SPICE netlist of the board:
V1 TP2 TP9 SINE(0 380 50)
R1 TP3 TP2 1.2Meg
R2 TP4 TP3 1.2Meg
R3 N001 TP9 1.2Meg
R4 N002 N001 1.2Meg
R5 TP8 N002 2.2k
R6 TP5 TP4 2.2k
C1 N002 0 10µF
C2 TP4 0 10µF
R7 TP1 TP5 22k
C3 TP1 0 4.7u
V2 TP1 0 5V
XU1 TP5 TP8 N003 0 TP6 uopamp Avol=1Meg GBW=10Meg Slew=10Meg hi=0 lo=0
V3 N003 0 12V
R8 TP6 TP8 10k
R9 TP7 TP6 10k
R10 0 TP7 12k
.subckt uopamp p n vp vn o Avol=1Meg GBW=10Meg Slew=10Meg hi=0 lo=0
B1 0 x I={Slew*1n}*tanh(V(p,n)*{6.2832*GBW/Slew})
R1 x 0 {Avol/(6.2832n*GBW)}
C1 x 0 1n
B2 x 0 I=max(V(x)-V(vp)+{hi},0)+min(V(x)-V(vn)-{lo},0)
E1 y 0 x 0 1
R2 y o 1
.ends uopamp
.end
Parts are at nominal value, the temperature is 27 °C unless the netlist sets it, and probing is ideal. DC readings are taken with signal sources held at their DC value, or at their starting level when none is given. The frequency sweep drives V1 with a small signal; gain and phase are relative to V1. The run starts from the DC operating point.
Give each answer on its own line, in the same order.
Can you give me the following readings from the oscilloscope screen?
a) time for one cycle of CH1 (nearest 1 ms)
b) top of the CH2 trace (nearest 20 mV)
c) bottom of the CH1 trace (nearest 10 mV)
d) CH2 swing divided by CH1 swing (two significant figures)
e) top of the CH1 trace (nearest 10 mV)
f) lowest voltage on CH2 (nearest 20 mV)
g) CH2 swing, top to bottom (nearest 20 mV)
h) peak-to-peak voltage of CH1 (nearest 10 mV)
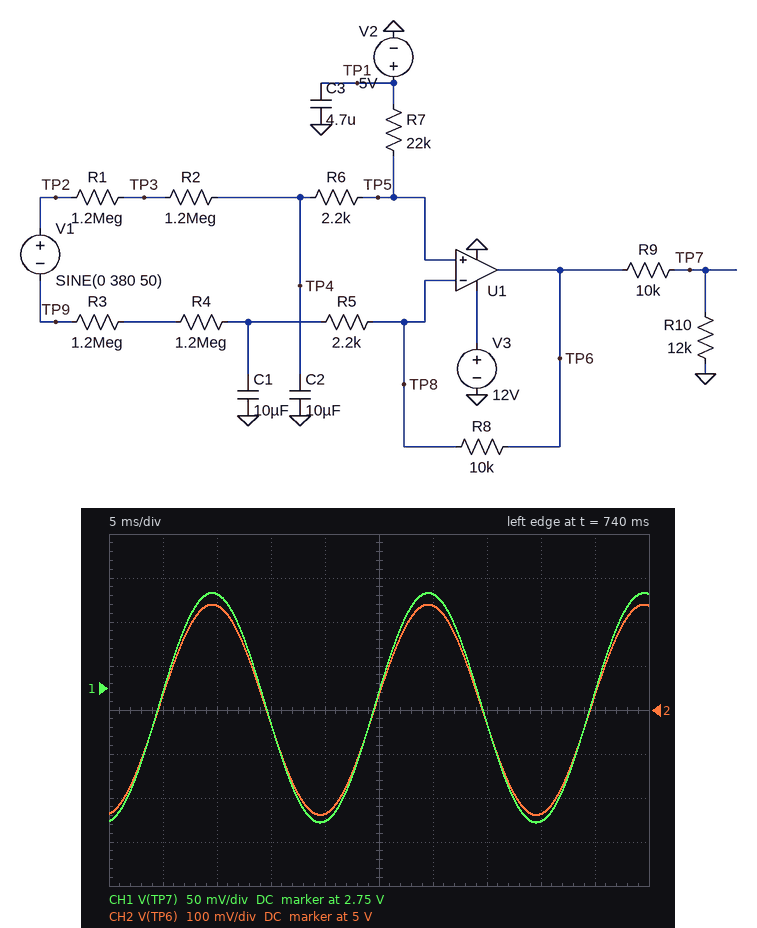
20 ms
5.24 V
2.60 V
1.8
2.86 V
4.76 V
480 mV
260 mV
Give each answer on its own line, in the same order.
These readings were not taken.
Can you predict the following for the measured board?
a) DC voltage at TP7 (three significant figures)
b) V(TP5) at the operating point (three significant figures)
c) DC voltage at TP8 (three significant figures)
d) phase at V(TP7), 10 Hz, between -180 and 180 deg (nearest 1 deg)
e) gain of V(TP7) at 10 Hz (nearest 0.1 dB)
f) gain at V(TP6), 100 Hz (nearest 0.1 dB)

2.73 V
5.00 V
5.00 V
-56 deg
-57.0 dB
-70.0 dB
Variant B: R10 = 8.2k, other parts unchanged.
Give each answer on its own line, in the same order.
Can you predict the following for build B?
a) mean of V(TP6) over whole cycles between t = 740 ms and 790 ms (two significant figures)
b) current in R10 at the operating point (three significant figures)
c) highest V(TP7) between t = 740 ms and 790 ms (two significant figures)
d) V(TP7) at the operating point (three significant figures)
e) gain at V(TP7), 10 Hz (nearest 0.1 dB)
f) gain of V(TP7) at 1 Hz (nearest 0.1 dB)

5.0 V
275 µA
2.4 V
2.25 V
-58.7 dB
-52.7 dB
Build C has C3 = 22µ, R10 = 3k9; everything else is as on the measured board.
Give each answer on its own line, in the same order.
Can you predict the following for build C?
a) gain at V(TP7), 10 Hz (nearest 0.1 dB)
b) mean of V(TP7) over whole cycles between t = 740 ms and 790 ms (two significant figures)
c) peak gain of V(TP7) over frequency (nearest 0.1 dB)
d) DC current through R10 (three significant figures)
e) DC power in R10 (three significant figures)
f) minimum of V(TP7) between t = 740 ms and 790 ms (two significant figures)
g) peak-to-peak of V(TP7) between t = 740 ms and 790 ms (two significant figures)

-62.8 dB
1.4 V
-54.6 dB
360 µA
505 µW
1.3 V
130 mV
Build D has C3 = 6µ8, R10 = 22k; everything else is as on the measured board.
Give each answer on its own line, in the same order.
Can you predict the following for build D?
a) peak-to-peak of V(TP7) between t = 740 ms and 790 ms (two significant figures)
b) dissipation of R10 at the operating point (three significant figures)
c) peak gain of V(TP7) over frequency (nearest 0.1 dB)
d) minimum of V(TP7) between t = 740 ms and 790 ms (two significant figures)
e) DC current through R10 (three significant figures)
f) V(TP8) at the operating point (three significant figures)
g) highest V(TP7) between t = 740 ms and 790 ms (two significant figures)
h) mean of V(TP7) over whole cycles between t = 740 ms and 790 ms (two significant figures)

330 mV
537 µW
-46.8 dB
3.3 V
156 µA
5.00 V
3.6 V
3.4 V
